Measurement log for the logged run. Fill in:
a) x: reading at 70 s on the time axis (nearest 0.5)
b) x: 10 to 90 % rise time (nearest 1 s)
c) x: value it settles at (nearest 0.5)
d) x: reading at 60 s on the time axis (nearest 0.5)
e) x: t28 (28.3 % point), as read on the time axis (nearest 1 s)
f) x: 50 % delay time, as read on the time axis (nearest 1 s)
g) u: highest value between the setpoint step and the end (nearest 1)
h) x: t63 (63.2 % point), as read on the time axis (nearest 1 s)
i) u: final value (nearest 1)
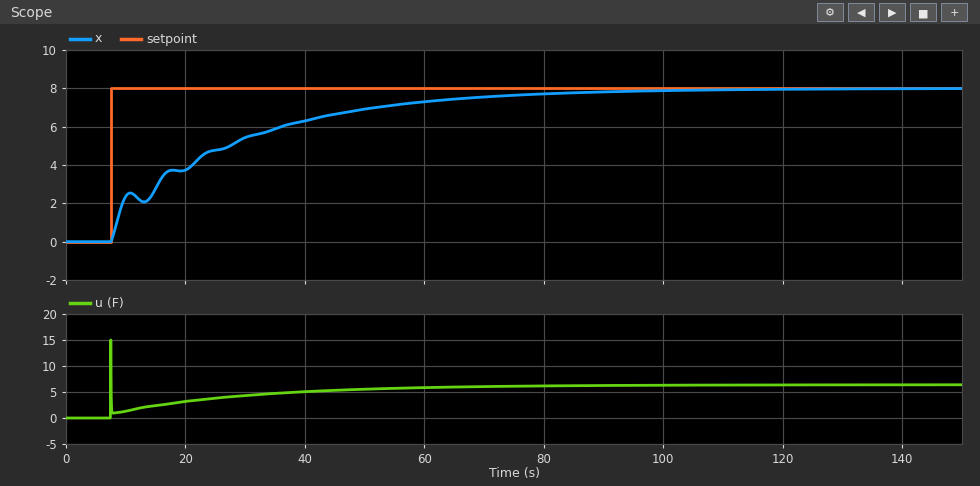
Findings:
7.5
49 s
8.0
7.5
10 s
21 s
15
28 s
6
